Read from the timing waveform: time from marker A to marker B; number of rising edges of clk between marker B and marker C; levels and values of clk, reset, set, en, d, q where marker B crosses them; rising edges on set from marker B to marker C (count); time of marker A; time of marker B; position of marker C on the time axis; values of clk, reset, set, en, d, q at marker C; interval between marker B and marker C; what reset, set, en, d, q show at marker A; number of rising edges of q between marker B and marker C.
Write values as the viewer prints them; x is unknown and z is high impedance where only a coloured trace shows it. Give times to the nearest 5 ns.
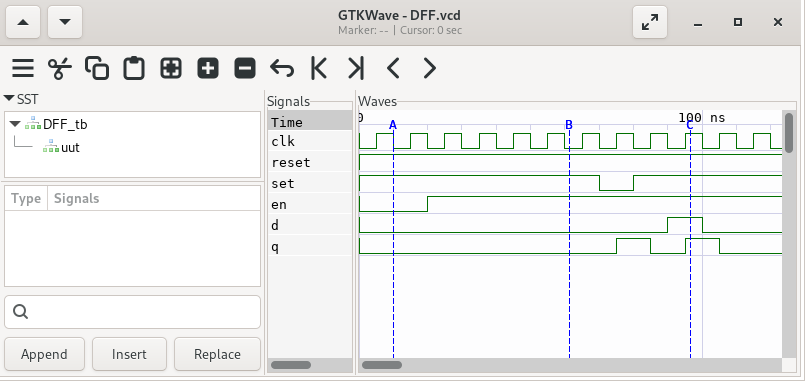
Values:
50 ns
4
clk=0, reset=1, set=1, en=1, d=0, q=0
1
10 ns
60 ns
95 ns
clk=1, reset=1, set=1, en=1, d=1, q=1
35 ns
reset=1, set=1, en=0, d=0, q=0
2
